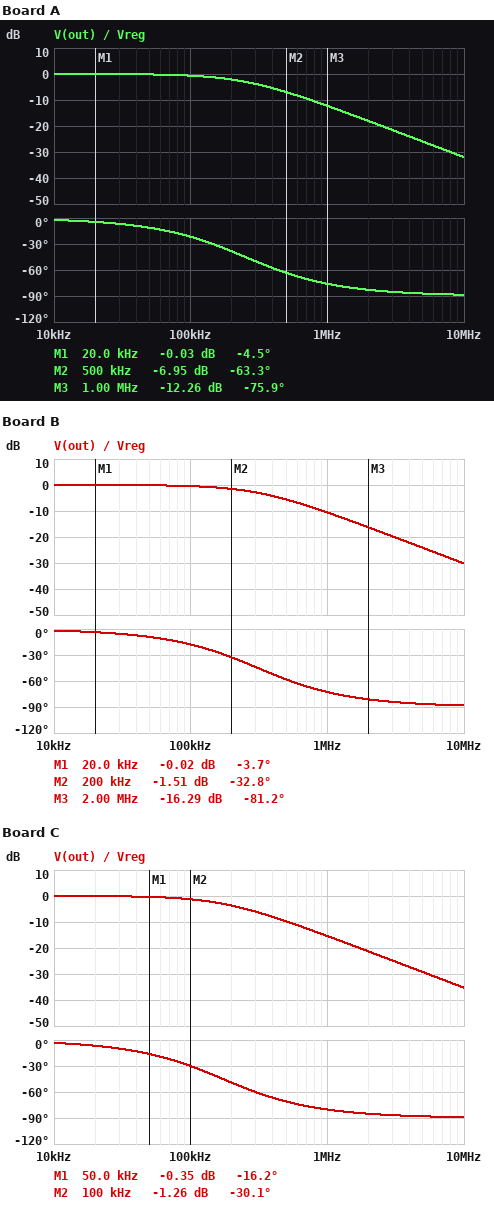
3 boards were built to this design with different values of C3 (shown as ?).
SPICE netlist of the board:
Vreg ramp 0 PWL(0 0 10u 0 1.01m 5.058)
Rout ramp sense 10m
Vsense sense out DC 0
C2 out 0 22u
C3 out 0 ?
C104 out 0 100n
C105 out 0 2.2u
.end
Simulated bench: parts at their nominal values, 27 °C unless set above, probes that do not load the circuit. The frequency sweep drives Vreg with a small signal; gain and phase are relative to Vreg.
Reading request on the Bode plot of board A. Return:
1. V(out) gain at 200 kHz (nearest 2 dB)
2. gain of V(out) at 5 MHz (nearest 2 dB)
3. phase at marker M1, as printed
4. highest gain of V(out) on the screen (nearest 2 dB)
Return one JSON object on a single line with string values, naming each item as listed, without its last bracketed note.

{"V(out) gain at 200 kHz": "-2 dB", "gain of V(out) at 5 MHz": "-26 dB", "phase at marker M1, as printed": "-4.5 deg", "highest gain of V(out) on the screen": "0 dB"}
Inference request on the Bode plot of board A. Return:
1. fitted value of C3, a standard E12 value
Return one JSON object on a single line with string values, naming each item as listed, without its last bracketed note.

{"fitted value of C3, a standard E12 value": "39 µF"}
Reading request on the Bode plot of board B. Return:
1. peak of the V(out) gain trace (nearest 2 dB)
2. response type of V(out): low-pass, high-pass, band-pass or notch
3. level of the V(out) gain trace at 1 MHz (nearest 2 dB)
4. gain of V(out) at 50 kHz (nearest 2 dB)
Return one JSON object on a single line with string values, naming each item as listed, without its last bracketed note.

{"peak of the V(out) gain trace": "0 dB", "response type of V(out): low-pass, high-pass, band-pass or notch": "low-pass", "level of the V(out) gain trace at 1 MHz": "-10 dB", "gain of V(out) at 50 kHz": "0 dB"}
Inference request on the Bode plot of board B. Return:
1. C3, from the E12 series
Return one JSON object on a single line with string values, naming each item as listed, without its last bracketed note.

{"C3, from the E12 series": "27 µF"}
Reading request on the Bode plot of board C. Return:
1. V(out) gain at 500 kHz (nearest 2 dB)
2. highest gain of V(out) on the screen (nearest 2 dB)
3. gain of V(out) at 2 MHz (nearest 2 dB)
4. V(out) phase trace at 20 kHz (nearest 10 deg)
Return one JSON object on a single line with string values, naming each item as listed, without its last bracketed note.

{"V(out) gain at 500 kHz": "-10 dB", "highest gain of V(out) on the screen": "0 dB", "gain of V(out) at 2 MHz": "-22 dB", "V(out) phase trace at 20 kHz": "-10 deg"}
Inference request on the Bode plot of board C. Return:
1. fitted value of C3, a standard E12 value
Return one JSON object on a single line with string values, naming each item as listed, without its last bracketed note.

{"fitted value of C3, a standard E12 value": "68 µF"}
